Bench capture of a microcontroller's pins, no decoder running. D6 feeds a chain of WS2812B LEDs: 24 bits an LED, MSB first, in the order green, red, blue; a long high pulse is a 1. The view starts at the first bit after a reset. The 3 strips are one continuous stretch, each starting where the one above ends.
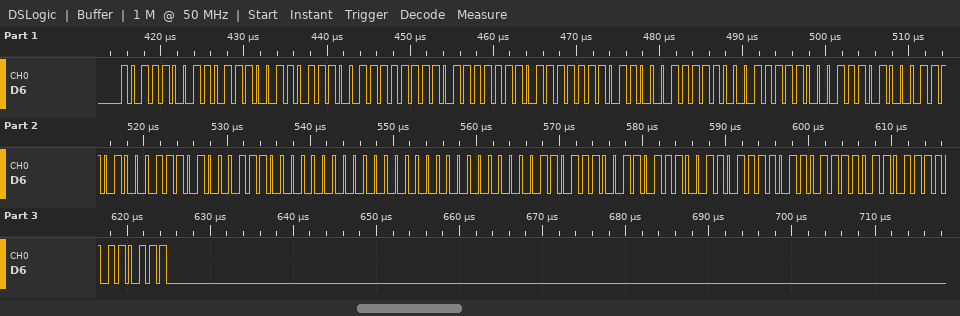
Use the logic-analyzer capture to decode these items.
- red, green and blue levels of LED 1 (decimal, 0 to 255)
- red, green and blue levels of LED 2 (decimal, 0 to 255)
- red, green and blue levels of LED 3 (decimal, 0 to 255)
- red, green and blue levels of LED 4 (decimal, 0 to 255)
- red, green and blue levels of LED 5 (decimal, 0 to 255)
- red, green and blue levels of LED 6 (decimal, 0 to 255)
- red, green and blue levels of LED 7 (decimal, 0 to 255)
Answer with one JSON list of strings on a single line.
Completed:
["185, 185, 185", "254, 254, 254", "199, 199, 199", "71, 71, 71", "0, 0, 0", "55, 55, 55", "183, 183, 183"]
